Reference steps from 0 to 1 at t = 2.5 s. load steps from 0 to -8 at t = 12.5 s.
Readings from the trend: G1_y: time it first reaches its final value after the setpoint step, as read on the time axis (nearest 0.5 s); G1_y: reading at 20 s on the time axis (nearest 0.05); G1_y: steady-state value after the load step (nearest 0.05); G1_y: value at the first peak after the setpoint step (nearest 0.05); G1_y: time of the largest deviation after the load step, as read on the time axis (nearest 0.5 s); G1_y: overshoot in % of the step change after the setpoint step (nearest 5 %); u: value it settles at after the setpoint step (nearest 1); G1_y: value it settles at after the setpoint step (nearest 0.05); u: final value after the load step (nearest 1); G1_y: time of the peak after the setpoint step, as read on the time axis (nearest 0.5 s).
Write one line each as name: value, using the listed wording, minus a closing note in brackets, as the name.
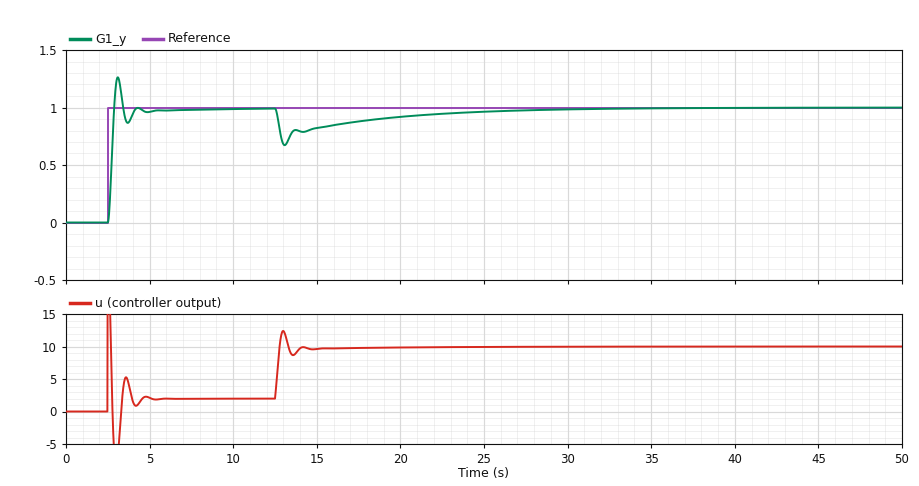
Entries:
G1_y: time it first reaches its final value after the setpoint step, as read on the time axis: 3.0 s
G1_y: reading at 20 s on the time axis: 0.90
G1_y: steady-state value after the load step: 1.00
G1_y: value at the first peak after the setpoint step: 1.25
G1_y: time of the largest deviation after the load step, as read on the time axis: 13.0 s
G1_y: overshoot in % of the step change after the setpoint step: 25 %
u: value it settles at after the setpoint step: 2
G1_y: value it settles at after the setpoint step: 1.00
u: final value after the load step: 10
G1_y: time of the peak after the setpoint step, as read on the time axis: 3.0 s
